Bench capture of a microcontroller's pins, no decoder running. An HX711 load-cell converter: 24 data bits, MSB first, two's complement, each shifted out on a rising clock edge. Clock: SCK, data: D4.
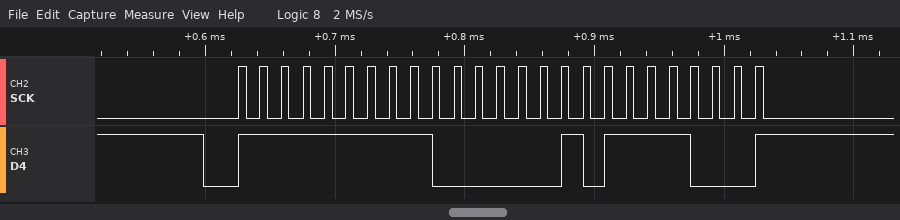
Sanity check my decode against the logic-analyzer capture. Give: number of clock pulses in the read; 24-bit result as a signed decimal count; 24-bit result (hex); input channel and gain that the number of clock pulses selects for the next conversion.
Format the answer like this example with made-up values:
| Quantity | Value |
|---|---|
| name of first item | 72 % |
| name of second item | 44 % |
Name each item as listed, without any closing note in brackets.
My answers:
| Quantity | Value |
|---|---|
| number of clock pulses in the read | 25 |
| 24-bit result as a signed decimal count | -32392 |
| 24-bit result | 0xFF8178 |
| input channel and gain that the number of clock pulses selects for the next conversion | channel A, gain 128 |
